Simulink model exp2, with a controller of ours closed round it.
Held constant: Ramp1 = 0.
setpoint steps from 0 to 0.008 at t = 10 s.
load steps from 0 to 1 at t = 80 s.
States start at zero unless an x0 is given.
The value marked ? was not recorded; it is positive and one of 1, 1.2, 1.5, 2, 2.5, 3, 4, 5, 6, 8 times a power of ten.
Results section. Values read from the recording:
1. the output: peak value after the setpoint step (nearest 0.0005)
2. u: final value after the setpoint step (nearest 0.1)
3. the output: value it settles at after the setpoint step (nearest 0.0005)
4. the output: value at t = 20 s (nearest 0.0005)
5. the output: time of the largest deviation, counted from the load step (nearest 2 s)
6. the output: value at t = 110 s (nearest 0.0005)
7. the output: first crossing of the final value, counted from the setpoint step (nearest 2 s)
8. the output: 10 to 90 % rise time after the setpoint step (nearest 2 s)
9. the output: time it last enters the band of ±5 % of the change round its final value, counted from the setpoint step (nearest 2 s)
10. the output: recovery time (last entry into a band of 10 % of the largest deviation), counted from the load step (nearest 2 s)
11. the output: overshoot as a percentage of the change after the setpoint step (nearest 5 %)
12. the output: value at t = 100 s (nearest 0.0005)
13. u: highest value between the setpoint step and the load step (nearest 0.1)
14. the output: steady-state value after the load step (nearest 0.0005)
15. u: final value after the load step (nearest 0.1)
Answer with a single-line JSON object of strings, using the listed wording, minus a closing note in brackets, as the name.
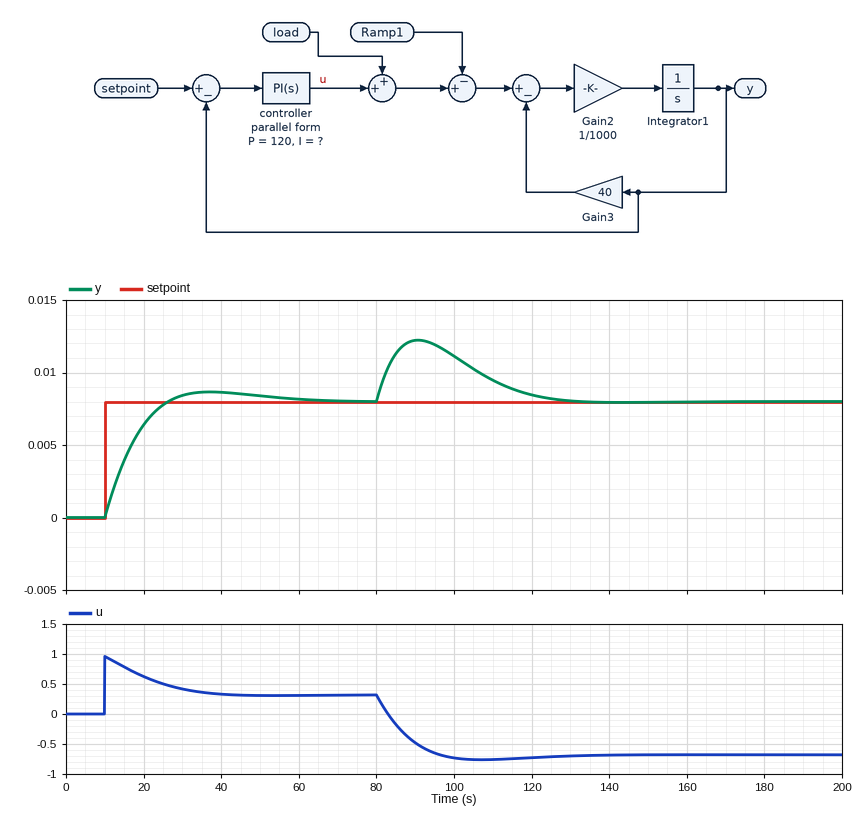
{"the output: peak value after the setpoint step": "0.0085", "u: final value after the setpoint step": "0.3", "the output: value it settles at after the setpoint step": "0.0080", "the output: value at t = 20 s": "0.0065", "the output: time of the largest deviation, counted from the load step": "10 s", "the output: value at t = 110 s": "0.0095", "the output: first crossing of the final value, counted from the setpoint step": "16 s", "the output: 10 to 90 % rise time after the setpoint step": "12 s", "the output: time it last enters the band of ±5 % of the change round its final value, counted from the setpoint step": "40 s", "the output: recovery time (last entry into a band of 10 % of the largest deviation), counted from the load step": "40 s", "the output: overshoot as a percentage of the change after the setpoint step": "10 %", "the output: value at t = 100 s": "0.0110", "u: highest value between the setpoint step and the load step": "1.0", "the output: steady-state value after the load step": "0.0080", "u: final value after the load step": "-0.7"}
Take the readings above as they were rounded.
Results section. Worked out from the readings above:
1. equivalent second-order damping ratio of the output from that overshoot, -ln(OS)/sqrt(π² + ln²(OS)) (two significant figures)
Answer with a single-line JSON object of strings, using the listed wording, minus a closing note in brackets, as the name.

{"equivalent second-order damping ratio of the output from that overshoot, -ln(OS)/sqrt(π² + ln²(OS))": "0.59"}
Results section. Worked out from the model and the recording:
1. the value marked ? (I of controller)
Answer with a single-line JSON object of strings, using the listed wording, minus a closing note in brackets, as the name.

{"the value marked ?": "10"}
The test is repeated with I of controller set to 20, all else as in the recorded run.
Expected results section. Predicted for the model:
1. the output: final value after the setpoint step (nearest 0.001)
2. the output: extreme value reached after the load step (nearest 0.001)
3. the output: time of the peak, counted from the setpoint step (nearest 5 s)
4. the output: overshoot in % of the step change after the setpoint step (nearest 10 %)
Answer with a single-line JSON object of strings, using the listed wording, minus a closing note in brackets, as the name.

{"the output: final value after the setpoint step": "0.008", "the output: extreme value reached after the load step": "0.012", "the output: time of the peak, counted from the setpoint step": "20 s", "the output: overshoot in % of the step change after the setpoint step": "20 %"}
